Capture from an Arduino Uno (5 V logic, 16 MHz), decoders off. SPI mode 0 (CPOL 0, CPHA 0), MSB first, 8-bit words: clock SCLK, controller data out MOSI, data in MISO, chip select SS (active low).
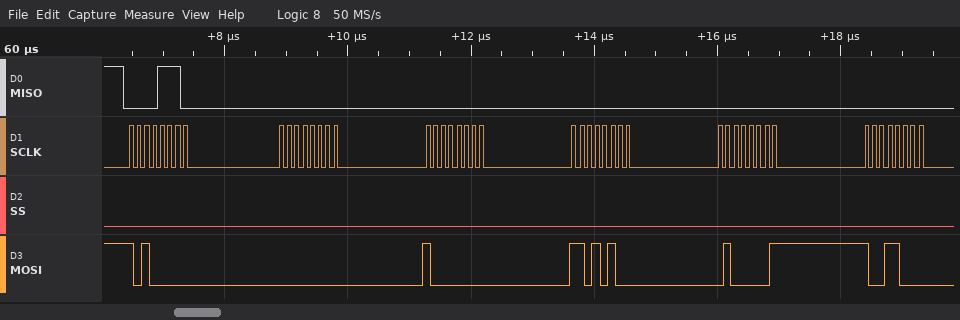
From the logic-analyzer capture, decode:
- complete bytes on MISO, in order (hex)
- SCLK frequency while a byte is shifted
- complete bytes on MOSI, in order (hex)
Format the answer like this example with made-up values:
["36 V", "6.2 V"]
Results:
["0E 00 00 00 00 00", "8 MHz", "A0 00 80 D4 41 98"]
